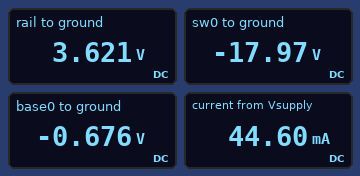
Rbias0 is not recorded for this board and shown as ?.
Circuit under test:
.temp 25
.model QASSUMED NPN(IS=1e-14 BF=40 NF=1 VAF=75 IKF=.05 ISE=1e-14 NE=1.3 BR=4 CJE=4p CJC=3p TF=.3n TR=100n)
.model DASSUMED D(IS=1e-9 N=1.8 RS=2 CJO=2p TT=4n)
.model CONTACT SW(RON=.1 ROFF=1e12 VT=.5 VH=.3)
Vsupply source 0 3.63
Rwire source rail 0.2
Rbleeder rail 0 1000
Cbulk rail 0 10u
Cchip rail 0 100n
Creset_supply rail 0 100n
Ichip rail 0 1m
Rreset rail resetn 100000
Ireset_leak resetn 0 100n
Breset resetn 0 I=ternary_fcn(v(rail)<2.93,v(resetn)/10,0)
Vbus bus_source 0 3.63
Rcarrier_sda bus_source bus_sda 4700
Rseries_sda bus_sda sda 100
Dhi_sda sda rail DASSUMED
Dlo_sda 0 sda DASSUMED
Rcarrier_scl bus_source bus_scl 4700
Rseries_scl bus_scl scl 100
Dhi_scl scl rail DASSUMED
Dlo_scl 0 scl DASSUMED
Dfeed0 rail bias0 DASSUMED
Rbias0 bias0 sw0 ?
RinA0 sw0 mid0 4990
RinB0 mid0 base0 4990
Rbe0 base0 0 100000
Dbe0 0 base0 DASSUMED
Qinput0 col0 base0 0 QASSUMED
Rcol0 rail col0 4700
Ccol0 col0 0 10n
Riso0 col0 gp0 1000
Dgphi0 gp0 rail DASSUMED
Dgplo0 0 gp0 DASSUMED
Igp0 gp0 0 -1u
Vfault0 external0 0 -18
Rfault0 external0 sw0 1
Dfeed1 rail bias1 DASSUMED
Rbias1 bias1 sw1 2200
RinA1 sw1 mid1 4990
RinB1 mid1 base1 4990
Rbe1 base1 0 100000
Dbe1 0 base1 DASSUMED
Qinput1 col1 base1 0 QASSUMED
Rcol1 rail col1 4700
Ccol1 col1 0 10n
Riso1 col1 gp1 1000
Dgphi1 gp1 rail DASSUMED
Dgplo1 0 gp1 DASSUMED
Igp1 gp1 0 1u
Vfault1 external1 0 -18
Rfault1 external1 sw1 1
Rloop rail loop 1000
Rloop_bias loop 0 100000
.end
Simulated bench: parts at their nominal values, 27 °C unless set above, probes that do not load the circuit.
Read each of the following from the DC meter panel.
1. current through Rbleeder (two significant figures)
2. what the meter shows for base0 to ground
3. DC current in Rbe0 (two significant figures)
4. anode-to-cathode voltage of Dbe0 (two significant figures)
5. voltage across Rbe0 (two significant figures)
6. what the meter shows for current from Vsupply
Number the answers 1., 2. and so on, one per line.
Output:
1. 3.6 mA
2. -0.676 V
3. 6.8 µA
4. 680 mV
5. 680 mV
6. 44.60 mA
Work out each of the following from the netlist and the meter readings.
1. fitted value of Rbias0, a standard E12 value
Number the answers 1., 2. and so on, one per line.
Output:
1. 680 Ω
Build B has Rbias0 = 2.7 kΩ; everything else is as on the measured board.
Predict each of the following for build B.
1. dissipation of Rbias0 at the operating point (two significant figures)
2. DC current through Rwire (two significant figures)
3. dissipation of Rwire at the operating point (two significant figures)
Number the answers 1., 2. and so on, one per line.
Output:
1. 160 mW
2. 22 mA
3. 96 µW
